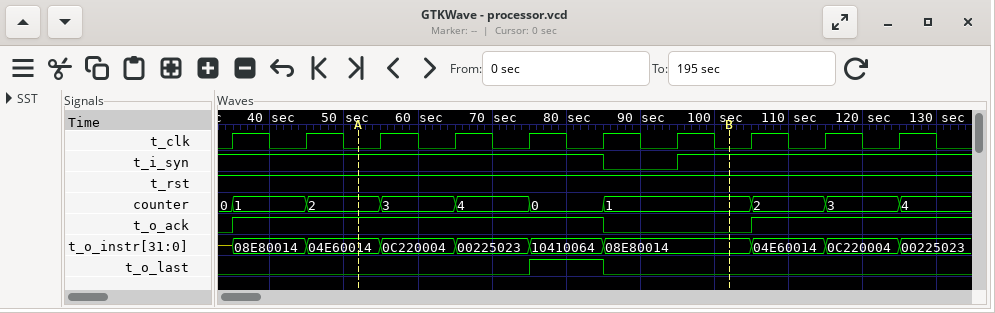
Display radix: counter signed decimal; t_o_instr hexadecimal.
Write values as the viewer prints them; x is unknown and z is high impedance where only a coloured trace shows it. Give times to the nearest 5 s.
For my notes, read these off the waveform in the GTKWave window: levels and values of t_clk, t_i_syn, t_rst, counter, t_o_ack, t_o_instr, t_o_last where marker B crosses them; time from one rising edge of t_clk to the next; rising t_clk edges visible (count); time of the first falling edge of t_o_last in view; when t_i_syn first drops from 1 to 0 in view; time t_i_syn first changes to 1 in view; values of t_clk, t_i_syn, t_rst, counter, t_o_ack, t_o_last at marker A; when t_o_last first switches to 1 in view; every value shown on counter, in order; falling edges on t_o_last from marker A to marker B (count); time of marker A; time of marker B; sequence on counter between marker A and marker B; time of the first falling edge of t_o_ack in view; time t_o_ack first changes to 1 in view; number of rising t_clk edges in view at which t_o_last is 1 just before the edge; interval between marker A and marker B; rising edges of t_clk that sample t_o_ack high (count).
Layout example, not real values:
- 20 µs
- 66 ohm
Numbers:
- t_clk=0, t_i_syn=1, t_rst=1, counter=1, t_o_ack=0, t_o_instr=08E80014, t_o_last=0
- 10 s
- 10
- 85 s
- 85 s
- 95 s
- t_clk=0, t_i_syn=1, t_rst=1, counter=2, t_o_ack=1, t_o_last=0
- 75 s
- 0, 1, 2, 3, 4, 0, 1, 2, 3, 4
- 1
- 50 s
- 100 s
- 2, 3, 4, 0, 1
- 85 s
- 35 s
- 1
- 50 s
- 7
